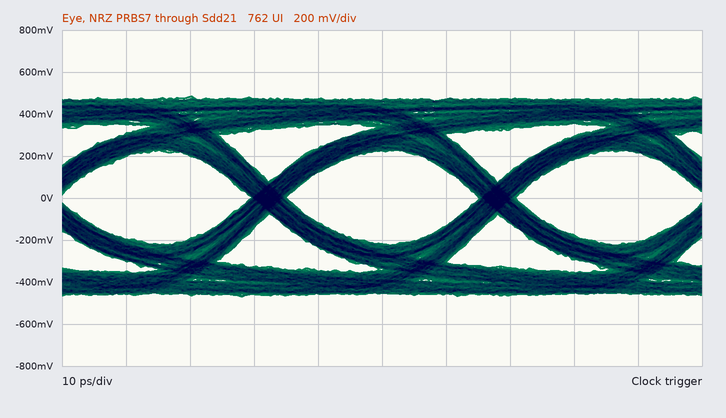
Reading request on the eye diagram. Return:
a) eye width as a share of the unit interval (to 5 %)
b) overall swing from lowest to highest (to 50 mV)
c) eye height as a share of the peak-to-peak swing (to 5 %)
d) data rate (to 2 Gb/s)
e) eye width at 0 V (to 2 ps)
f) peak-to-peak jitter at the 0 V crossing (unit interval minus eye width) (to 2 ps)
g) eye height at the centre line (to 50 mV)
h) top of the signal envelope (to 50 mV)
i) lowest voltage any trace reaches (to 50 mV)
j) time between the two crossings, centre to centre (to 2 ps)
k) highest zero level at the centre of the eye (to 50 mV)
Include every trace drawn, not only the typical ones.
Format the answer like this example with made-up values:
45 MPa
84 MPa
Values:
85 %
950 mV
45 %
28 Gb/s
30 ps
6 ps
450 mV
500 mV
-450 mV
36 ps
-200 mV
